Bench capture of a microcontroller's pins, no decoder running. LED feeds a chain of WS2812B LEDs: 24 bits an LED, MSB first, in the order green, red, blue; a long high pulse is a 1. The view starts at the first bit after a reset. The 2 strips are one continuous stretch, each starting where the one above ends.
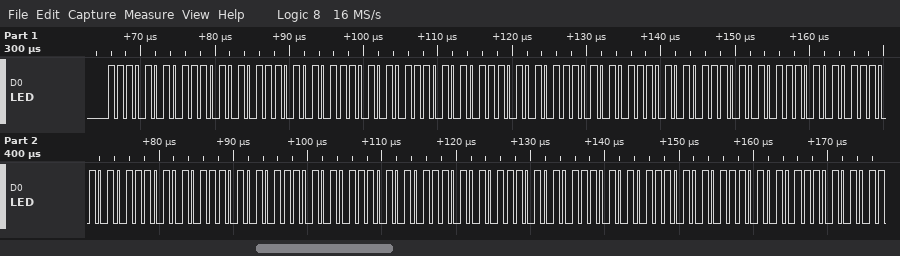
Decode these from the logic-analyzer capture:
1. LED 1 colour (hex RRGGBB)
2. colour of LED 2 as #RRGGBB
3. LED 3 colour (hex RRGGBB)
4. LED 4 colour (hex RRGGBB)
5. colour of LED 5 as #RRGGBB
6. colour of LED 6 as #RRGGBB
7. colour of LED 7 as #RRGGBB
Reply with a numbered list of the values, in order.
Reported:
1. #EAEAEA
2. #EAEAEA
3. #EAEAEA
4. #EAEAEA
5. #EAEAEA
6. #EAEAEA
7. #EAEAEA
